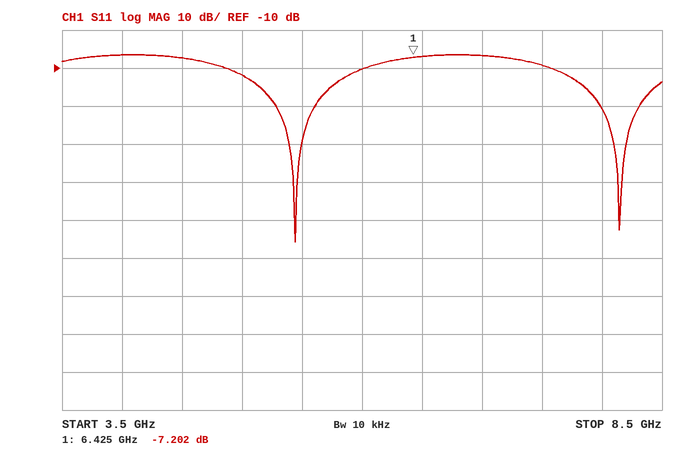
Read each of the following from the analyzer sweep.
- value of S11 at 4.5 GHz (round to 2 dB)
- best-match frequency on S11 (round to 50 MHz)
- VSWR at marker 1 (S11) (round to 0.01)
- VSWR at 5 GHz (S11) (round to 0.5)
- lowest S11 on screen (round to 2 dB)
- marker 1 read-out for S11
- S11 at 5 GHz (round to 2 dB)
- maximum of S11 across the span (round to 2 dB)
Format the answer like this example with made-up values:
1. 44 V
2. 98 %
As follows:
1. -8 dB
2. 5.45 GHz
3. 2.55
4. 1.5
5. -56 dB
6. -7.202 dB
7. -12 dB
8. -6 dB
